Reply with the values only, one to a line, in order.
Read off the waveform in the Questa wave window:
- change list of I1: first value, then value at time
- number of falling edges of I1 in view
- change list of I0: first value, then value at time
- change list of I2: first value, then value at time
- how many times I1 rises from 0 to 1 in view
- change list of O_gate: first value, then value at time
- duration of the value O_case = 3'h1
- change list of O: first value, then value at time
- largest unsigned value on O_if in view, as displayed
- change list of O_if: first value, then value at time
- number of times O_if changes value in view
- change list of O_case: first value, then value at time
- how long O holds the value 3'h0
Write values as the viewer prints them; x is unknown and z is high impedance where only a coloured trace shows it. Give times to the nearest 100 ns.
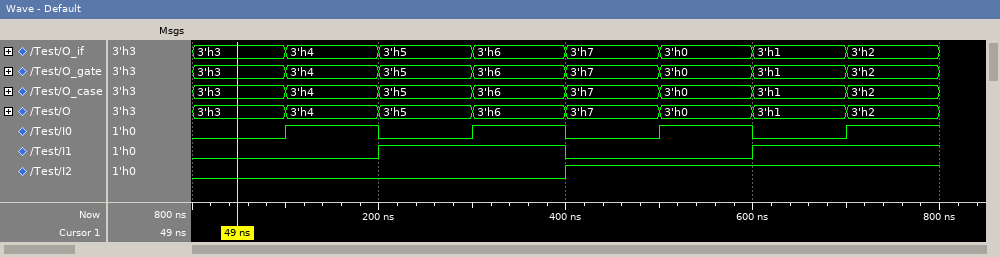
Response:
0, 1 at 200 ns, 0 at 400 ns, 1 at 600 ns
1
0, 1 at 100 ns, 0 at 200 ns, 1 at 300 ns, 0 at 400 ns, 1 at 500 ns, 0 at 600 ns, 1 at 700 ns
0, 1 at 400 ns
2
3'h3, 3'h4 at 100 ns, 3'h5 at 200 ns, 3'h6 at 300 ns, 3'h7 at 400 ns, 3'h0 at 500 ns, 3'h1 at 600 ns, 3'h2 at 700 ns
100 ns
3'h3, 3'h4 at 100 ns, 3'h5 at 200 ns, 3'h6 at 300 ns, 3'h7 at 400 ns, 3'h0 at 500 ns, 3'h1 at 600 ns, 3'h2 at 700 ns
3'h7
3'h3, 3'h4 at 100 ns, 3'h5 at 200 ns, 3'h6 at 300 ns, 3'h7 at 400 ns, 3'h0 at 500 ns, 3'h1 at 600 ns, 3'h2 at 700 ns
7
3'h3, 3'h4 at 100 ns, 3'h5 at 200 ns, 3'h6 at 300 ns, 3'h7 at 400 ns, 3'h0 at 500 ns, 3'h1 at 600 ns, 3'h2 at 700 ns
100 ns
